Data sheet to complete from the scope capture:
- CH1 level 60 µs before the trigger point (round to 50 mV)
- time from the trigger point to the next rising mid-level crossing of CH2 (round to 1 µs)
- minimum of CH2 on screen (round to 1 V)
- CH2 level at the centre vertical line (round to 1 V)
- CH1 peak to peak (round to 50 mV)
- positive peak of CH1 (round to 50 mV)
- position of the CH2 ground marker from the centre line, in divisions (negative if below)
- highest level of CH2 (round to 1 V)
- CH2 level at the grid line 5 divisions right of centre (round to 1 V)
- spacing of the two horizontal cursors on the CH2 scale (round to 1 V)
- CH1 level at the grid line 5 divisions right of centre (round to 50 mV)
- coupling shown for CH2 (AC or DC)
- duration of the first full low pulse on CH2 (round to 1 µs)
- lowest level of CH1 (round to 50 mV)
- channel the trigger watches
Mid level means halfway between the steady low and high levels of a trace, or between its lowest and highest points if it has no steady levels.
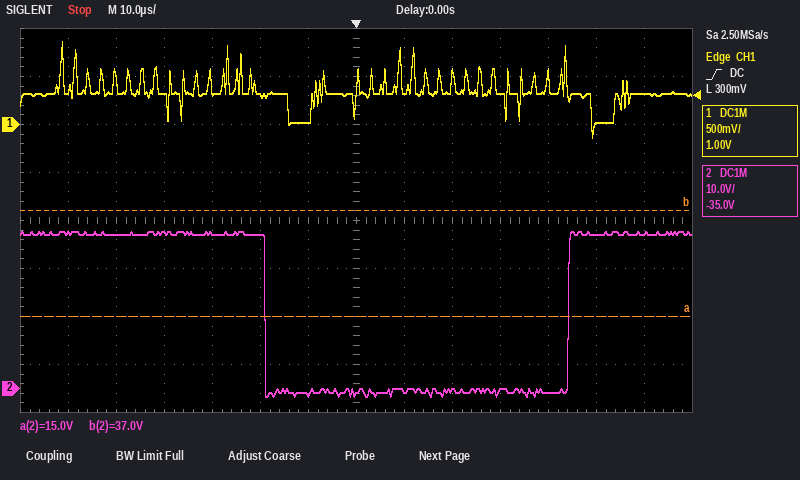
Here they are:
350 mV
44 µs
-2 V
-1 V
1.00 V
850 mV
-3.5 div
33 V
32 V
22 V
0 mV
DC
63 µs
-150 mV
CH1
